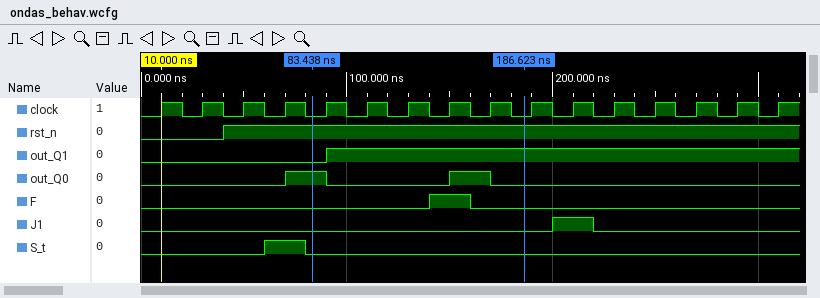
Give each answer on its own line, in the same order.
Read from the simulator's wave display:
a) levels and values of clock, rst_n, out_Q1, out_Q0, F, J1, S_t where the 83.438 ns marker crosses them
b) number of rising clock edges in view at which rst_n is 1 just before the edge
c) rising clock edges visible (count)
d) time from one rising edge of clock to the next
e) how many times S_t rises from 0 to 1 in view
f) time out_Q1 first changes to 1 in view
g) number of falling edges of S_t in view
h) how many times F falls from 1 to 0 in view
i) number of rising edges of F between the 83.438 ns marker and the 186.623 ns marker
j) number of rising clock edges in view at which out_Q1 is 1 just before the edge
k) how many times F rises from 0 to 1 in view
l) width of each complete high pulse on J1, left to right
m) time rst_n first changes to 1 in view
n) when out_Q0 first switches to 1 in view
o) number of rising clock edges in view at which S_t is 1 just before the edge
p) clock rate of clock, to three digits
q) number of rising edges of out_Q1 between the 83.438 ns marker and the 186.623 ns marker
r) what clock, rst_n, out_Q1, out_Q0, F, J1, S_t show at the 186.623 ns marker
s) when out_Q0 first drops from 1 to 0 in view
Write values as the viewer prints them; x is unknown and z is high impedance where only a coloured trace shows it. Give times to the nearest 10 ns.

clock=0, rst_n=1, out_Q1=0, out_Q0=1, F=0, J1=0, S_t=0
14
16
20 ns
1
90 ns
1
1
1
11
1
20 ns
40 ns
70 ns
1
50.0 MHz
1
clock=0, rst_n=1, out_Q1=1, out_Q0=0, F=0, J1=0, S_t=0
90 ns
